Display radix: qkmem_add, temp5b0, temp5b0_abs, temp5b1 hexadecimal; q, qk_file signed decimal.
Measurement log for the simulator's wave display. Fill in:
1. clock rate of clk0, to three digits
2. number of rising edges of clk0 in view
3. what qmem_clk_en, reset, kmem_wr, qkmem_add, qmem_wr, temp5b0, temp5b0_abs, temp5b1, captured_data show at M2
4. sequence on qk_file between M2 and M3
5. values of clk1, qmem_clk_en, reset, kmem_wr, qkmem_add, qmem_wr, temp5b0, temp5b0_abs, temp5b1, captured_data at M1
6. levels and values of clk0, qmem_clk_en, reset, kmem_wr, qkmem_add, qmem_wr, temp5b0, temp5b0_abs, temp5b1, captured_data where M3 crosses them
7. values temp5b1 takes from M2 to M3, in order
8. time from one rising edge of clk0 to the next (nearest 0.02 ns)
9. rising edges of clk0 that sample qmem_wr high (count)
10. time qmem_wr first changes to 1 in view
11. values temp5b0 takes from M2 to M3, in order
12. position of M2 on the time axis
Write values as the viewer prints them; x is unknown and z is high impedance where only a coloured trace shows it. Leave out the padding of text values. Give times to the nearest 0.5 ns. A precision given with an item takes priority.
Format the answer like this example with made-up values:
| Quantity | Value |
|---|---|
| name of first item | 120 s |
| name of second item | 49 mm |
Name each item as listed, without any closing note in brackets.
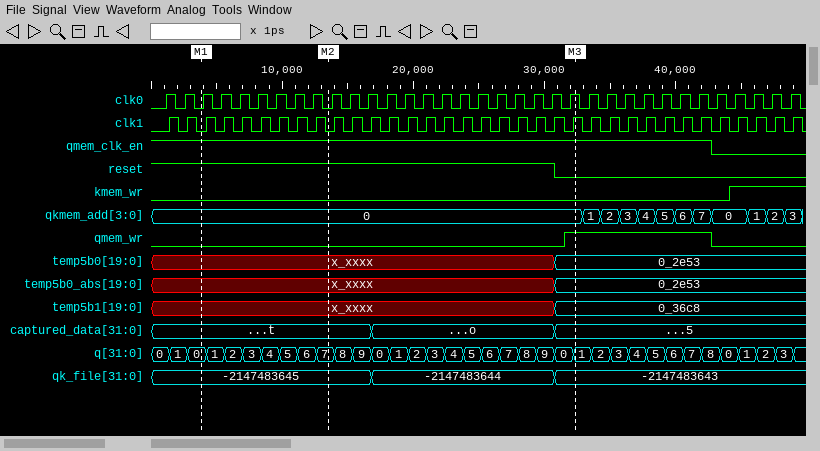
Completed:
| Quantity | Value |
|---|---|
| clock rate of clk0, to three digits | 714 MHz |
| number of rising edges of clk0 in view | 35 |
| what qmem_clk_en, reset, kmem_wr, qkmem_add, qmem_wr, temp5b0, temp5b0_abs, temp5b1, captured_data show at M2 | qmem_clk_en=1, reset=1, kmem_wr=0, qkmem_add=0, qmem_wr=0, temp5b0=x_xxxx, temp5b0_abs=x_xxxx, temp5b1=x_xxxx, captured_data=t |
| sequence on qk_file between M2 and M3 | -2147483645, -2147483644, -2147483643 |
| values of clk1, qmem_clk_en, reset, kmem_wr, qkmem_add, qmem_wr, temp5b0, temp5b0_abs, temp5b1, captured_data at M1 | clk1=0, qmem_clk_en=1, reset=1, kmem_wr=0, qkmem_add=0, qmem_wr=0, temp5b0=x_xxxx, temp5b0_abs=x_xxxx, temp5b1=x_xxxx, captured_data=t |
| levels and values of clk0, qmem_clk_en, reset, kmem_wr, qkmem_add, qmem_wr, temp5b0, temp5b0_abs, temp5b1, captured_data where M3 crosses them | clk0=1, qmem_clk_en=1, reset=0, kmem_wr=0, qkmem_add=0, qmem_wr=1, temp5b0=0_2e53, temp5b0_abs=0_2e53, temp5b1=0_36c8, captured_data=5 |
| values temp5b1 takes from M2 to M3, in order | x_xxxx, 0_36c8 |
| time from one rising edge of clk0 to the next | 1.4 ns |
| rising edges of clk0 that sample qmem_wr high | 8 |
| time qmem_wr first changes to 1 in view | 31.5 ns |
| values temp5b0 takes from M2 to M3, in order | x_xxxx, 0_2e53 |
| position of M2 on the time axis | 13.5 ns |
